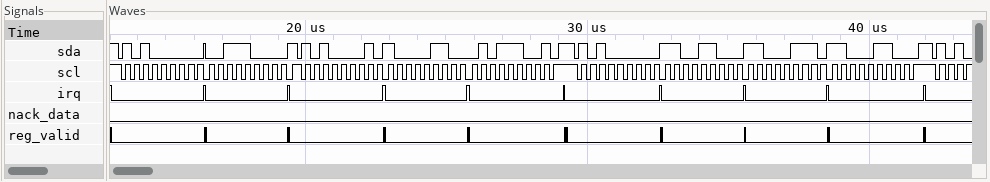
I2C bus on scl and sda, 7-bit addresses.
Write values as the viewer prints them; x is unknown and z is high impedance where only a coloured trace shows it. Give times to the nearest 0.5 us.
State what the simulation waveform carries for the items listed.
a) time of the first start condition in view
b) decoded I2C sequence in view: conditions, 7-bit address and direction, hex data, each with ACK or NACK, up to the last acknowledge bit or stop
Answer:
13.5 us
start, address 50 write ACK, 38 ACK, repeated start, address 50 read ACK, 86 ACK, 5C NACK, stop, start, address 50 write ACK, CC ACK, C7 ACK, C6 ACK, stop
